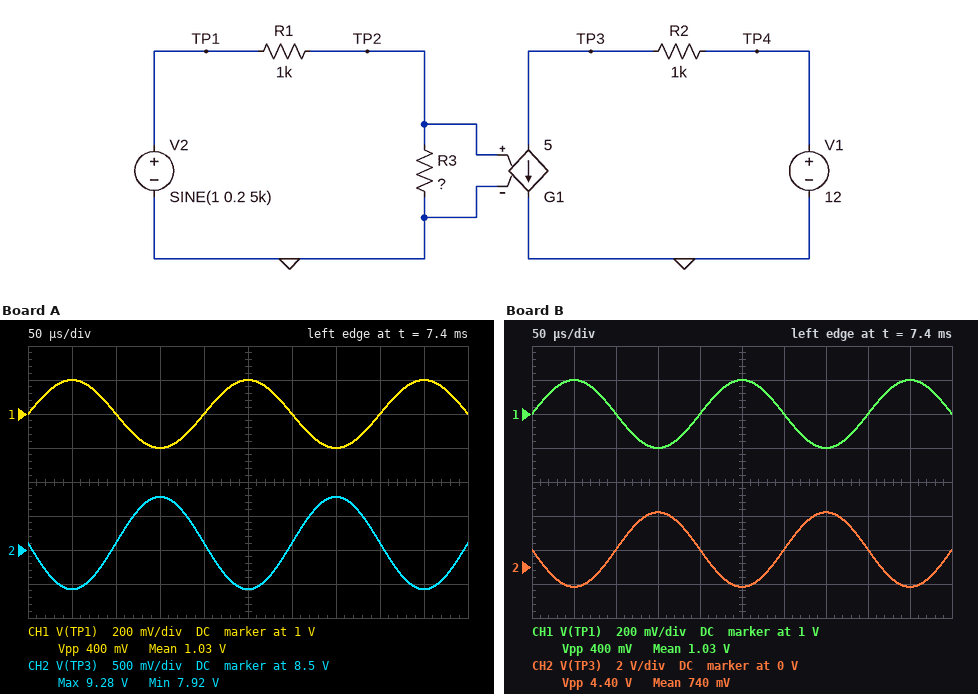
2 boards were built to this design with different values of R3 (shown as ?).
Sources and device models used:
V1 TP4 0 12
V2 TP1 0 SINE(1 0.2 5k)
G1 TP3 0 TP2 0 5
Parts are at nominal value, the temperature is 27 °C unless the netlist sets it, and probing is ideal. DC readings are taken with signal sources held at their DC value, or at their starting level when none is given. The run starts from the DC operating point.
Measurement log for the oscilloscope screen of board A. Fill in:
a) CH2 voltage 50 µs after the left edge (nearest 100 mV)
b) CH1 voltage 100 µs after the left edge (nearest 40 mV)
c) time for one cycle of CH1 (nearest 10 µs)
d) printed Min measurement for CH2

7.9 V
1.00 V
200 µs
7.92 V
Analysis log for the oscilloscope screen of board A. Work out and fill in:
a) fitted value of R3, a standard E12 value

0.68 Ω
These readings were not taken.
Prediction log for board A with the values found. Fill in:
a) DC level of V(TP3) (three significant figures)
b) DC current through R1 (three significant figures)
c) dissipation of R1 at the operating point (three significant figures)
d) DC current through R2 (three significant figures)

8.60 V
999 µA
999 µW
3.40 mA
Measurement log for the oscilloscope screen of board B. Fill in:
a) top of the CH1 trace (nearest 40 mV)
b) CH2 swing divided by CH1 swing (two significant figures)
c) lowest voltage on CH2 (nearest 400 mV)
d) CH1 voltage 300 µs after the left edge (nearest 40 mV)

1.20 V
11
-1.2 V
1.00 V
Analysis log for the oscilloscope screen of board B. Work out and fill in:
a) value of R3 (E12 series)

2.2 Ω
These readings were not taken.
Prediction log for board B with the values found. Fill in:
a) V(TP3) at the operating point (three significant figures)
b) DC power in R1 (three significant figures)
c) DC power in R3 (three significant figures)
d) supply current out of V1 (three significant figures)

1.02 V
996 µW
2.19 µW
11.0 mA
